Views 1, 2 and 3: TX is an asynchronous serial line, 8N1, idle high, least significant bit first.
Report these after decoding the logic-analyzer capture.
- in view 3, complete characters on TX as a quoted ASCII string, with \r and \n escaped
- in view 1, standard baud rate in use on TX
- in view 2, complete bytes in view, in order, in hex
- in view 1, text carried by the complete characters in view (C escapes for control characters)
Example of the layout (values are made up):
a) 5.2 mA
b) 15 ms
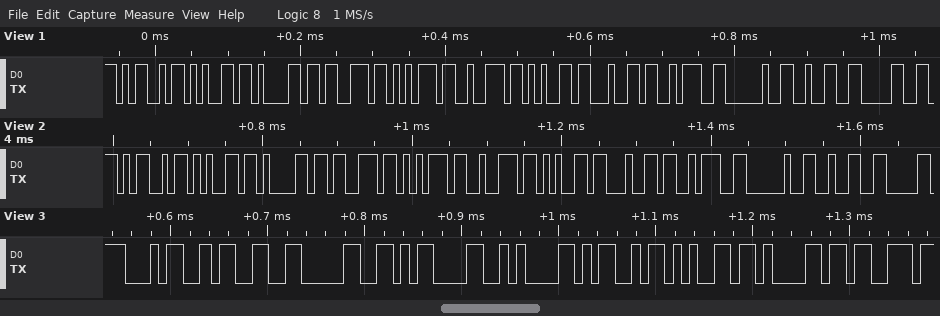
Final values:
a) "430\r\nMeas"
b) 115200 baud
c) 0x4D 0x65 0x61 0x73 0x75 0x72 0x65 0x64 0x3A 0x20 0x32
d) "Measured: 20"
